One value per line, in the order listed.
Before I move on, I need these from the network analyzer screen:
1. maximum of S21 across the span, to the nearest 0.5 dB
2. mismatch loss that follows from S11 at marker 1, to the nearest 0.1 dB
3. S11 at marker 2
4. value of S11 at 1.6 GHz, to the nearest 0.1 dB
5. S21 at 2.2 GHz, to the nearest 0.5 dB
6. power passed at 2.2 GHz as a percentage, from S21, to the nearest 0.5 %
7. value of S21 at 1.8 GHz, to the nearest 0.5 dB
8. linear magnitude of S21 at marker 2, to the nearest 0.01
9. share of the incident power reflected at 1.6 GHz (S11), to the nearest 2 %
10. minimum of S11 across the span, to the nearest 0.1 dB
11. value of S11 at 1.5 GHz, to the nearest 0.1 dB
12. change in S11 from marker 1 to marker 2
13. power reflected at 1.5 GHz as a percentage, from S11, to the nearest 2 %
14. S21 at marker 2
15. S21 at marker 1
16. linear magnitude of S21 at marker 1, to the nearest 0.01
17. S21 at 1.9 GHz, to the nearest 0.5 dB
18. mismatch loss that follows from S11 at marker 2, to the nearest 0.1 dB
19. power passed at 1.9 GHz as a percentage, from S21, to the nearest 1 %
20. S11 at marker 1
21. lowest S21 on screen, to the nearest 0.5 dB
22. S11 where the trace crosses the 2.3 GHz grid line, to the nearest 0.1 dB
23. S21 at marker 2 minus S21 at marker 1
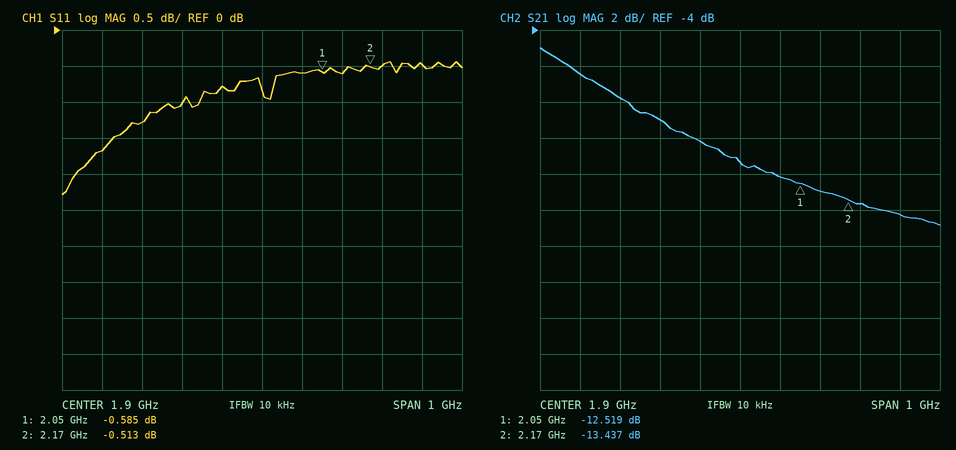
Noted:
-5.0 dB
9.0 dB
-0.513 dB
-1.3 dB
-13.5 dB
4.5 %
-10.0 dB
0.21
74 %
-2.3 dB
-1.7 dB
0.072 dB
68 %
-13.437 dB
-12.519 dB
0.24
-11.5 dB
9.5 dB
7 %
-0.585 dB
-15.0 dB
-0.5 dB
-0.918 dB
